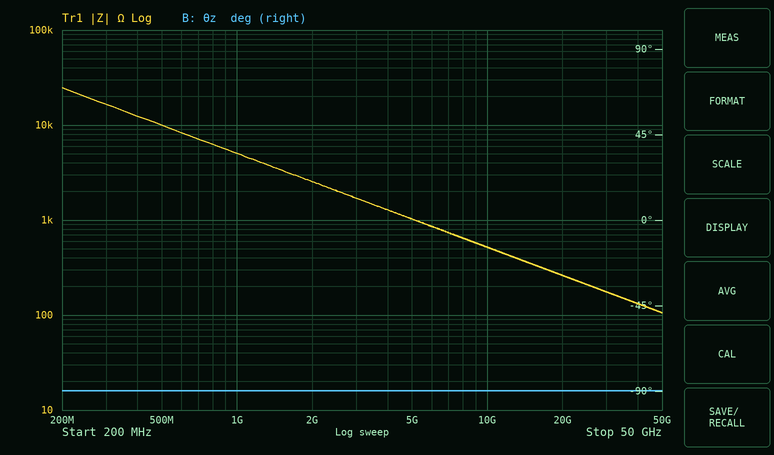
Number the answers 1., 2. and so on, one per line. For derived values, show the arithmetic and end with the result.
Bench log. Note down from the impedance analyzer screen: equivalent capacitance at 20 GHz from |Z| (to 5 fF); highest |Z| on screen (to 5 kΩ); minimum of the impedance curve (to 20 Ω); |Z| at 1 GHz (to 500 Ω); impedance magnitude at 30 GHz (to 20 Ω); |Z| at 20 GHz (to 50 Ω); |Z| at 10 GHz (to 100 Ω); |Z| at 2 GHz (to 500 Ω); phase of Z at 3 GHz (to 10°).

1. C = 1/(2π × 20 GHz × 250 Ω) ≈ 31.8 fF, so 30 fF to the nearest 5 fF
2. 25 kΩ
3. 100 Ω
4. 5.0 kΩ
5. 180 Ω
6. 250 Ω
7. 500 Ω
8. 2.5 kΩ
9. -90°
